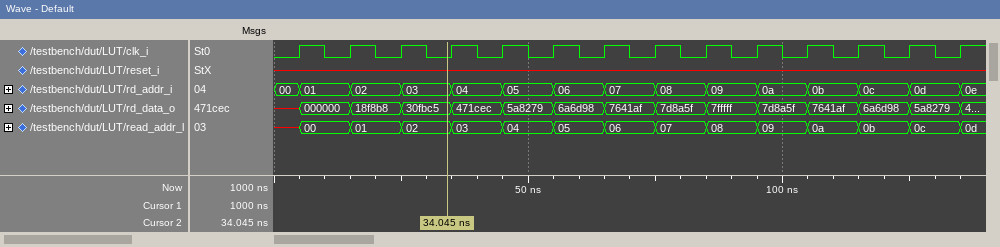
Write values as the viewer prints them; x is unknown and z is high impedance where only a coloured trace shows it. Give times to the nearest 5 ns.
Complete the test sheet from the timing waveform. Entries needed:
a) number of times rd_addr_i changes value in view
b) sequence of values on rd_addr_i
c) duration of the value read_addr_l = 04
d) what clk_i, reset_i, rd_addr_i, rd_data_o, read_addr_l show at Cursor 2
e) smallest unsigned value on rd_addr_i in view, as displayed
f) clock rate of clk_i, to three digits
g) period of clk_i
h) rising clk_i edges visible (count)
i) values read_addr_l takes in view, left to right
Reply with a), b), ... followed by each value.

a) 14
b) 00, 01, 02, 03, 04, 05, 06, 07, 08, 09, 0a, 0b, 0c, 0d, 0e
c) 10 ns
d) clk_i=0, reset_i=x, rd_addr_i=03, rd_data_o=30fbc5, read_addr_l=02
e) 00
f) 100 MHz
g) 10 ns
h) 14
i) x, 00, 01, 02, 03, 04, 05, 06, 07, 08, 09, 0a, 0b, 0c, 0d
